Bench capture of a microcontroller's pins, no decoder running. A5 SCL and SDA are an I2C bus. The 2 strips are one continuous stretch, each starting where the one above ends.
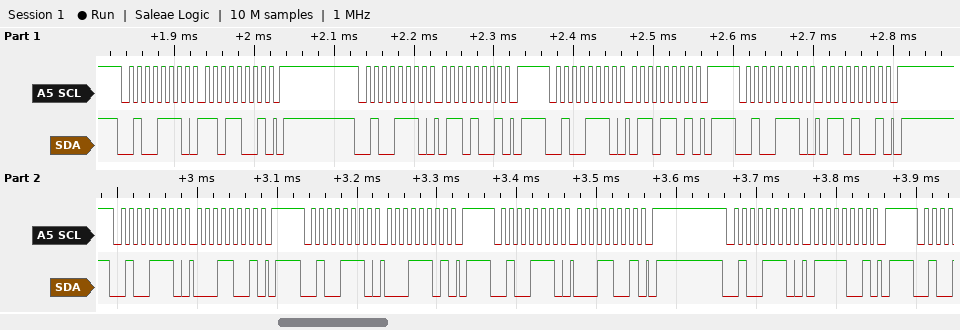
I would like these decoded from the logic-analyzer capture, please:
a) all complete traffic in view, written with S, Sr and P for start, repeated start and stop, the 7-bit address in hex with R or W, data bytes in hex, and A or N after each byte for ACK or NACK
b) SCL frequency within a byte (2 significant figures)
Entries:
S 27W A D9 A P S 27W A 69 A P S 27W A 6D A P S 27W A 69 A P S 27W A 19 A P S 27W A 1D A P S 27W A 19 A P S 27W A 79 A P
100 kHz
